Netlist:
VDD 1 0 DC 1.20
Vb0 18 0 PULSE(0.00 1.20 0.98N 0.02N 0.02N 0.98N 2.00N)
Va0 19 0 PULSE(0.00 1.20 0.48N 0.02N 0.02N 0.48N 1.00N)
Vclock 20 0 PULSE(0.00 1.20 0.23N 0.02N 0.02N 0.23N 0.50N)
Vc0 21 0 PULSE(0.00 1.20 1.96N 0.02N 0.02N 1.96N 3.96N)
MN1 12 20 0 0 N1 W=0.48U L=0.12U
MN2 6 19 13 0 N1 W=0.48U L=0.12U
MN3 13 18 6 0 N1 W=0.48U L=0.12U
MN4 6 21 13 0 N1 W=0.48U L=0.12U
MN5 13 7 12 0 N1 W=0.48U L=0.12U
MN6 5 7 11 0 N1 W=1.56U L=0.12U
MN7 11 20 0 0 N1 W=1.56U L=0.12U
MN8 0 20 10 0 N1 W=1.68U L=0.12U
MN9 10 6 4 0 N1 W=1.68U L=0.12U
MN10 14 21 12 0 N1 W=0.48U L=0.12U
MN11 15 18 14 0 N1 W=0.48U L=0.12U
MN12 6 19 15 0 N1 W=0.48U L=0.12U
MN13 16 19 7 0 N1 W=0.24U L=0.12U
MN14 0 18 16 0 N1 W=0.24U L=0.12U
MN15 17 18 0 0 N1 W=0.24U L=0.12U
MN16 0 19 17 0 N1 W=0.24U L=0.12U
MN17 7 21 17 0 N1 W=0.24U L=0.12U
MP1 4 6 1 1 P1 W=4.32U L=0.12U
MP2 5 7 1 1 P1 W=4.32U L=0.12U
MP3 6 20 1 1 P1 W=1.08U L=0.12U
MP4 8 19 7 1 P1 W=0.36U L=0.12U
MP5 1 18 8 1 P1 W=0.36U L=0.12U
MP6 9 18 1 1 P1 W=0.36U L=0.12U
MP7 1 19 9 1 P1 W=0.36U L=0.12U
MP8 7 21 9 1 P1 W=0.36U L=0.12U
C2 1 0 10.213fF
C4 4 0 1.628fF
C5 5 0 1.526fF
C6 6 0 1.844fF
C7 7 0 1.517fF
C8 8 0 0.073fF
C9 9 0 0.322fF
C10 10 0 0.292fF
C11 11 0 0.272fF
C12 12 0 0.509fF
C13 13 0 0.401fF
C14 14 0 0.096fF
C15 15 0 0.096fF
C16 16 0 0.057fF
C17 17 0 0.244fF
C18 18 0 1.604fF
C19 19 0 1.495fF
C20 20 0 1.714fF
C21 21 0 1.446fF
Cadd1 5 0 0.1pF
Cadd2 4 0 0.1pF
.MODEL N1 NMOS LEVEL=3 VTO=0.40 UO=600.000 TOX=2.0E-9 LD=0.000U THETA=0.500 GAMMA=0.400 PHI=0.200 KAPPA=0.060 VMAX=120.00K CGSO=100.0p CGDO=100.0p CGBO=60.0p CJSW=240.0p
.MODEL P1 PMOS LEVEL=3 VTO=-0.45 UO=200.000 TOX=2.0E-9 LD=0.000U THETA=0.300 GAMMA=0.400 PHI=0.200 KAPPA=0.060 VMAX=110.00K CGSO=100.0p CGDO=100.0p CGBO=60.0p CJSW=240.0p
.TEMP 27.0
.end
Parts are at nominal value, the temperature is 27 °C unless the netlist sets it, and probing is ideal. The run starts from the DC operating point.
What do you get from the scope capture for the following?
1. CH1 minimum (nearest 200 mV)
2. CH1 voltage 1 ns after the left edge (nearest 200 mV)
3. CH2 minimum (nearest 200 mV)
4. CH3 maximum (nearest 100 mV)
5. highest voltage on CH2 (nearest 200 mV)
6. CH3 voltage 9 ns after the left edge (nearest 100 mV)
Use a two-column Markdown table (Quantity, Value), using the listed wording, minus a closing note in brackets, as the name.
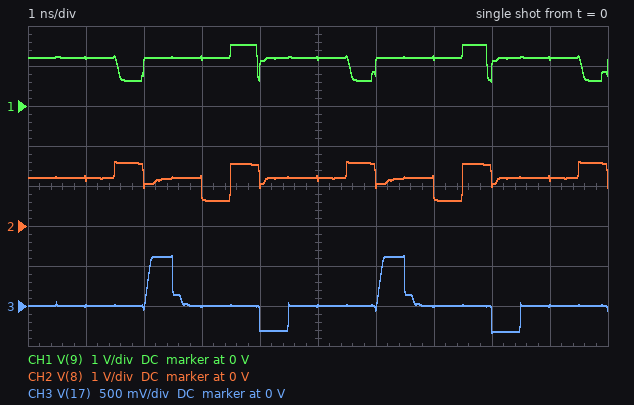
| Quantity | Value |
|---|---|
| CH1 minimum | 600 mV |
| CH1 voltage 1 ns after the left edge | 1.2 V |
| CH2 minimum | 600 mV |
| CH3 maximum | 600 mV |
| highest voltage on CH2 | 1.6 V |
| CH3 voltage 9 ns after the left edge | 0 V |
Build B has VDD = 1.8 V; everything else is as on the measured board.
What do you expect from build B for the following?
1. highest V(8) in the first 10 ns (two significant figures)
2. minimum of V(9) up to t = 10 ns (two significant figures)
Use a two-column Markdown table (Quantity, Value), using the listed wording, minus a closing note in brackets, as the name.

| Quantity | Value |
|---|---|
| highest V(8) in the first 10 ns | 1.9 V |
| minimum of V(9) up to t = 10 ns | 900 mV |
